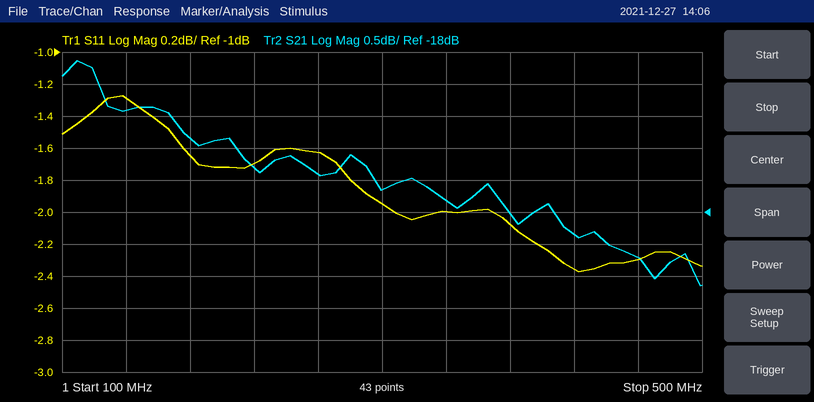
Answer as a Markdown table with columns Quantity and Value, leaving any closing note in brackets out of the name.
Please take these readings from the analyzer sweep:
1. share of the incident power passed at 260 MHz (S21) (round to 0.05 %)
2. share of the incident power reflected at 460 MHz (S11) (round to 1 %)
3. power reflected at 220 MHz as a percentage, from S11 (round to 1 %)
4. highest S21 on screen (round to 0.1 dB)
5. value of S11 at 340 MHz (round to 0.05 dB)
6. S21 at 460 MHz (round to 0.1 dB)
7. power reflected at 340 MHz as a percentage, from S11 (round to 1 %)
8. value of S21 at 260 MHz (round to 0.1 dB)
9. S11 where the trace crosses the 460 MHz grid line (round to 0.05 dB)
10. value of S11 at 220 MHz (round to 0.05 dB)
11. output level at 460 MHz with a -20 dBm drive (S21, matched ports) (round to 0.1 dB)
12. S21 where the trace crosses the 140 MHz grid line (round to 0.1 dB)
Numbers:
| Quantity | Value |
|---|---|
| share of the incident power passed at 260 MHz (S21) | 1.80 % |
| share of the incident power reflected at 460 MHz (S11) | 59 % |
| power reflected at 220 MHz as a percentage, from S11 | 68 % |
| highest S21 on screen | -15.6 dB |
| value of S11 at 340 MHz | -2.00 dB |
| S21 at 460 MHz | -18.7 dB |
| power reflected at 340 MHz as a percentage, from S11 | 63 % |
| value of S21 at 260 MHz | -17.4 dB |
| S11 where the trace crosses the 460 MHz grid line | -2.30 dB |
| value of S11 at 220 MHz | -1.70 dB |
| output level at 460 MHz with a -20 dBm drive (S21, matched ports) | -38.7 dBm |
| S21 where the trace crosses the 140 MHz grid line | -16.4 dB |
